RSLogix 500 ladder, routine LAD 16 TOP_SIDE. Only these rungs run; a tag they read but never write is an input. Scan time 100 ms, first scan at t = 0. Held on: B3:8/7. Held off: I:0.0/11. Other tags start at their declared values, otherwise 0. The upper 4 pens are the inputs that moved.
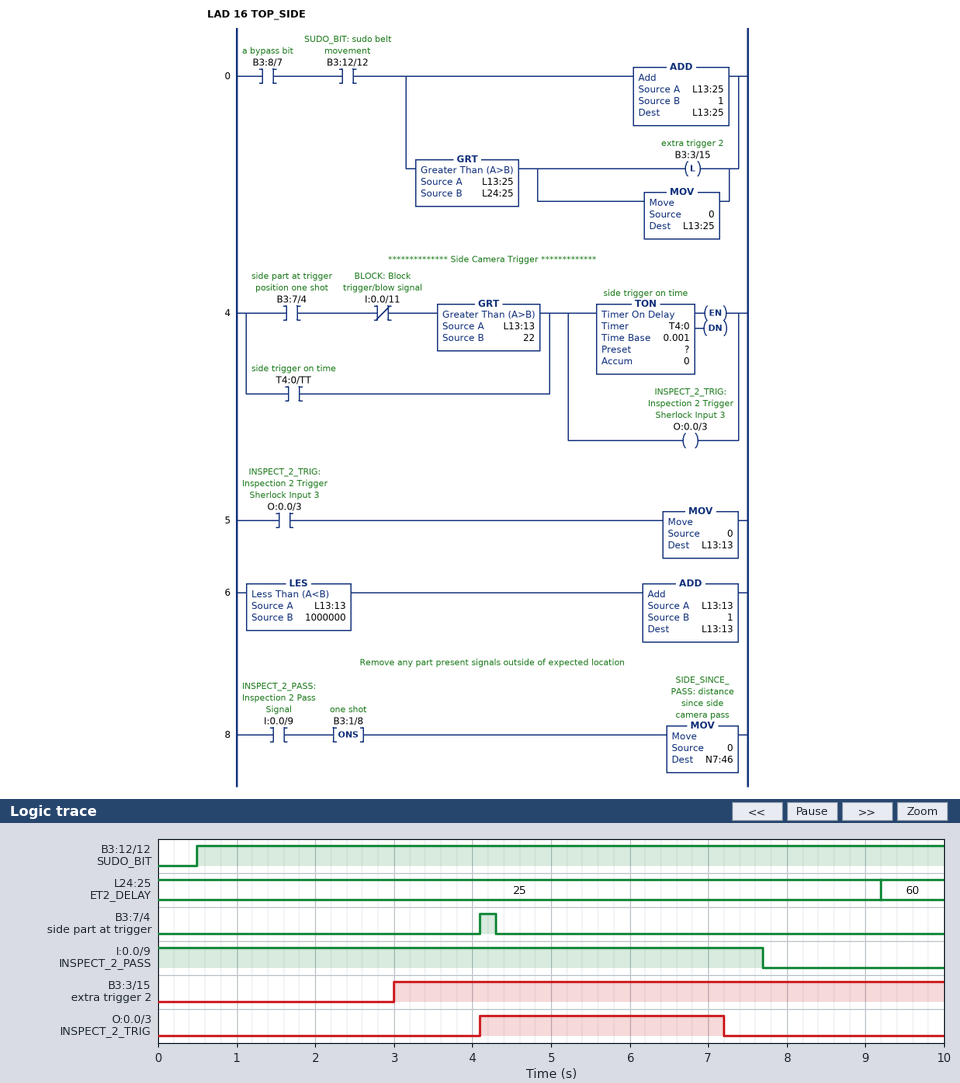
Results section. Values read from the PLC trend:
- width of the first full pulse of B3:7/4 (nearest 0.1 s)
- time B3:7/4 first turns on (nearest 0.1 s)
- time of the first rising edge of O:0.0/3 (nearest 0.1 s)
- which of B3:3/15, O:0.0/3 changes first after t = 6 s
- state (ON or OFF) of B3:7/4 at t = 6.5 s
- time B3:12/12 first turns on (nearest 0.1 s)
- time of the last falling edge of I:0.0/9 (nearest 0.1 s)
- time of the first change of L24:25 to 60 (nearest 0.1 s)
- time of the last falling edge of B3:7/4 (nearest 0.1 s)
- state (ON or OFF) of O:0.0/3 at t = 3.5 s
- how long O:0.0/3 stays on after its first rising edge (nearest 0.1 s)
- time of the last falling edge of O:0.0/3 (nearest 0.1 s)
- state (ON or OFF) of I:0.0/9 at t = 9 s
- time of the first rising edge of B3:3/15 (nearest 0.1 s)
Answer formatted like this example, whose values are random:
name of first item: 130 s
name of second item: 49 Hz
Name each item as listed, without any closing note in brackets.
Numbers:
width of the first full pulse of B3:7/4: 0.2 s
time B3:7/4 first turns on: 4.1 s
time of the first rising edge of O:0.0/3: 4.1 s
which of B3:3/15, O:0.0/3 changes first after t = 6 s: O:0.0/3
state (ON or OFF) of B3:7/4 at t = 6.5 s: OFF
time B3:12/12 first turns on: 0.5 s
time of the last falling edge of I:0.0/9: 7.7 s
time of the first change of L24:25 to 60: 9.2 s
time of the last falling edge of B3:7/4: 4.3 s
state (ON or OFF) of O:0.0/3 at t = 3.5 s: OFF
how long O:0.0/3 stays on after its first rising edge: 3.1 s
time of the last falling edge of O:0.0/3: 7.2 s
state (ON or OFF) of I:0.0/9 at t = 9 s: OFF
time of the first rising edge of B3:3/15: 3.0 s
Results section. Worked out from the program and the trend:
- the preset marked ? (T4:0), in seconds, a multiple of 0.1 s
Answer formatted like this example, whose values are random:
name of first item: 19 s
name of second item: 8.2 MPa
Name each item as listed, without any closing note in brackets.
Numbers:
the preset marked ? (T4:0), in seconds, a multiple of 0.1 s: 3.0 s
